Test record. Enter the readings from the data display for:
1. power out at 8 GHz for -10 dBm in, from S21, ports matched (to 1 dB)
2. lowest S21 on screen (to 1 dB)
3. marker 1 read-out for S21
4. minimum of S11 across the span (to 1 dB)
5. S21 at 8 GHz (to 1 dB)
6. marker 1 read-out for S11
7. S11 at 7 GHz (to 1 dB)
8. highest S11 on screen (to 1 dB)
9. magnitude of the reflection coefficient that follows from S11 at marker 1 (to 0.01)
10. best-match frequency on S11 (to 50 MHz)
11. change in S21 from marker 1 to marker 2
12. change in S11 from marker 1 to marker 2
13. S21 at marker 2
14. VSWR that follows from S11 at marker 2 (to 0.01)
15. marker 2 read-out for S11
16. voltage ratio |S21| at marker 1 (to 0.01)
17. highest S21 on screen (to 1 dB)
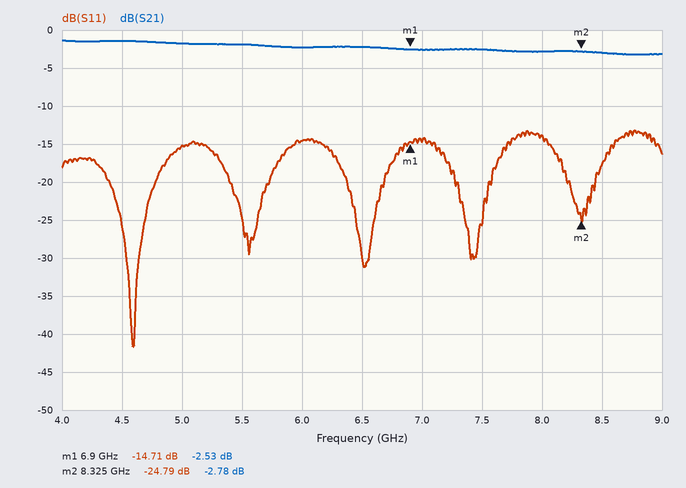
-13 dBm
-3 dB
-2.53 dB
-42 dB
-3 dB
-14.71 dB
-15 dB
-13 dB
0.18
4.60 GHz
-0.25 dB
-10.08 dB
-2.78 dB
1.12
-24.79 dB
0.75
-1 dB
